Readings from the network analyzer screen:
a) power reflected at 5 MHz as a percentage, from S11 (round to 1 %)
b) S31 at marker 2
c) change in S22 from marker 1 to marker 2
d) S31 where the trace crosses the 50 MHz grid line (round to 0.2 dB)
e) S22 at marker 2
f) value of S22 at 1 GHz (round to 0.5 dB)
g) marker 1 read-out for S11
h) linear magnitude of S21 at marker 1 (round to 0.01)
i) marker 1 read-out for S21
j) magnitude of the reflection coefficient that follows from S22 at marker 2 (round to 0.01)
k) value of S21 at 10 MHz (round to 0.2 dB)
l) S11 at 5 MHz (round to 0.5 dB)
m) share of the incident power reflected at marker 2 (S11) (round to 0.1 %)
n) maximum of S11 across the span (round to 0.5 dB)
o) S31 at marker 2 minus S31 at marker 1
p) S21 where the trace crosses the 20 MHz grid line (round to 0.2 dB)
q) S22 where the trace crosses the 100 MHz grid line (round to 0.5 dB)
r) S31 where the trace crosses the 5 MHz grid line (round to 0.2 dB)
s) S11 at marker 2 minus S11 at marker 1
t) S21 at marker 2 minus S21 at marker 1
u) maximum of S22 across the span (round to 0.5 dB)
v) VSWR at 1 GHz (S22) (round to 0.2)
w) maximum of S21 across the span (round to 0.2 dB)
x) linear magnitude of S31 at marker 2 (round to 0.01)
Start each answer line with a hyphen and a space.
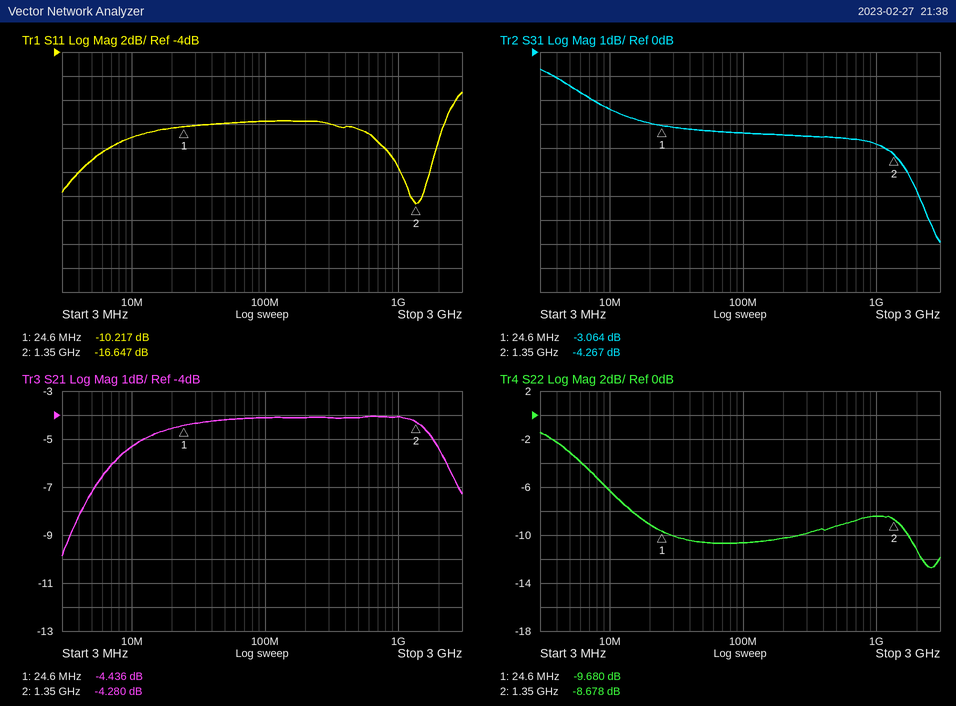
- 5 %
- -4.267 dB
- 1.002 dB
- -3.2 dB
- -8.678 dB
- -8.5 dB
- -10.217 dB
- 0.60
- -4.436 dB
- 0.37
- -5.4 dB
- -13.0 dB
- 2.2 %
- -7.5 dB
- -1.203 dB
- -4.6 dB
- -10.5 dB
- -1.4 dB
- -6.430 dB
- 0.156 dB
- -1.5 dB
- 2.2
- -4.0 dB
- 0.61
